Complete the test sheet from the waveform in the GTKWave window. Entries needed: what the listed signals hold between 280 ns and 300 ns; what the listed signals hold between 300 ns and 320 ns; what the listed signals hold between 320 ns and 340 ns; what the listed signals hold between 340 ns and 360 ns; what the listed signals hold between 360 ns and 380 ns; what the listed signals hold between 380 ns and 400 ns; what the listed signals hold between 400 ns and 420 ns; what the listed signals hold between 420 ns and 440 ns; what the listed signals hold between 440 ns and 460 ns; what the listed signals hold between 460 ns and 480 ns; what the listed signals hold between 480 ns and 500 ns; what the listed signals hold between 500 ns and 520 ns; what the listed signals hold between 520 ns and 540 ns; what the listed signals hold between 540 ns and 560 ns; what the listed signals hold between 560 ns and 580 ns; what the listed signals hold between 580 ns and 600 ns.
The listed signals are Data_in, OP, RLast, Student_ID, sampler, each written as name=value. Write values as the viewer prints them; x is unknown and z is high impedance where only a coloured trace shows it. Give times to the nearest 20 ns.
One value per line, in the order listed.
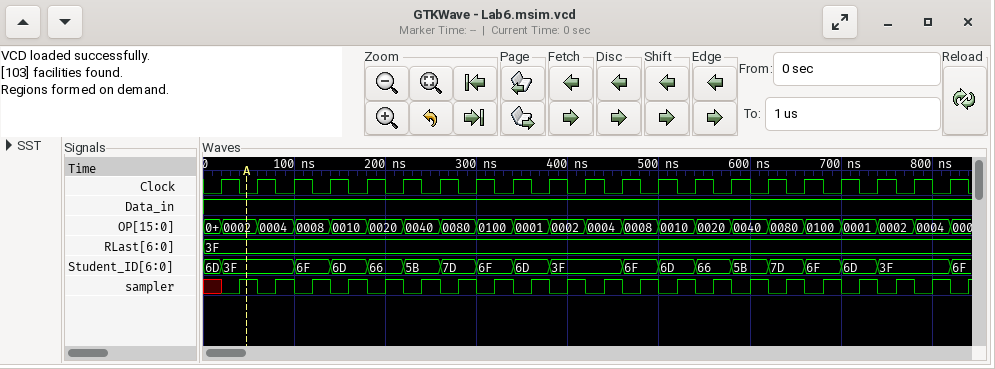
Data_in=1, OP=0080, RLast=3F, Student_ID=7D, sampler=1
Data_in=1, OP=0100, RLast=3F, Student_ID=6F, sampler=0
Data_in=1, OP=0100, RLast=3F, Student_ID=6F, sampler=1
Data_in=1, OP=0001, RLast=3F, Student_ID=6D, sampler=0
Data_in=1, OP=0001, RLast=3F, Student_ID=6D, sampler=1
Data_in=1, OP=0002, RLast=3F, Student_ID=3F, sampler=0
Data_in=1, OP=0002, RLast=3F, Student_ID=3F, sampler=1
Data_in=1, OP=0004, RLast=3F, Student_ID=3F, sampler=0
Data_in=1, OP=0004, RLast=3F, Student_ID=3F, sampler=1
Data_in=1, OP=0008, RLast=3F, Student_ID=6F, sampler=0
Data_in=1, OP=0008, RLast=3F, Student_ID=6F, sampler=1
Data_in=1, OP=0010, RLast=3F, Student_ID=6D, sampler=0
Data_in=1, OP=0010, RLast=3F, Student_ID=6D, sampler=1
Data_in=1, OP=0020, RLast=3F, Student_ID=66, sampler=0
Data_in=1, OP=0020, RLast=3F, Student_ID=66, sampler=1
Data_in=1, OP=0040, RLast=3F, Student_ID=5B, sampler=0
